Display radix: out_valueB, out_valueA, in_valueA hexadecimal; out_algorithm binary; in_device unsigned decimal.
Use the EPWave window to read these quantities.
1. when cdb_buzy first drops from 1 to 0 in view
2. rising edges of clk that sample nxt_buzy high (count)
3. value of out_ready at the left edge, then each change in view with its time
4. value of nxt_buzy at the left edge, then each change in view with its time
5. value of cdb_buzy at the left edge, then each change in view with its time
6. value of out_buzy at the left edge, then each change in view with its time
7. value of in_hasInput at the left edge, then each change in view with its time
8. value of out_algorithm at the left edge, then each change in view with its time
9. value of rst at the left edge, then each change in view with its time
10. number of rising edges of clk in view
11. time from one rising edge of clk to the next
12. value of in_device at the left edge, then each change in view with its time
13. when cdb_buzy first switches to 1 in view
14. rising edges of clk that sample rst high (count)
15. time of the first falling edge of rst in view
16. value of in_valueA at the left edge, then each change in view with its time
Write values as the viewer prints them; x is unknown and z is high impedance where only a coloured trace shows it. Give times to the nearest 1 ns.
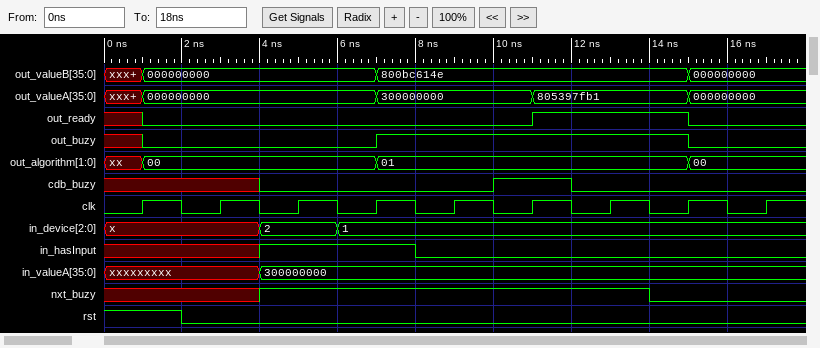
12 ns
5
x, 0 at 1 ns, 1 at 11 ns, 0 at 15 ns
x, 1 at 4 ns, 0 at 14 ns
x, 0 at 4 ns, 1 at 10 ns, 0 at 12 ns
x, 0 at 1 ns, 1 at 7 ns, 0 at 15 ns
x, 1 at 4 ns, 0 at 8 ns
xx, 00 at 1 ns, 01 at 7 ns, 00 at 15 ns
1, 0 at 2 ns
9
2 ns
x, 2 at 4 ns, 1 at 6 ns
10 ns
1
2 ns
xxxxxxxxx, 300000000 at 4 ns
